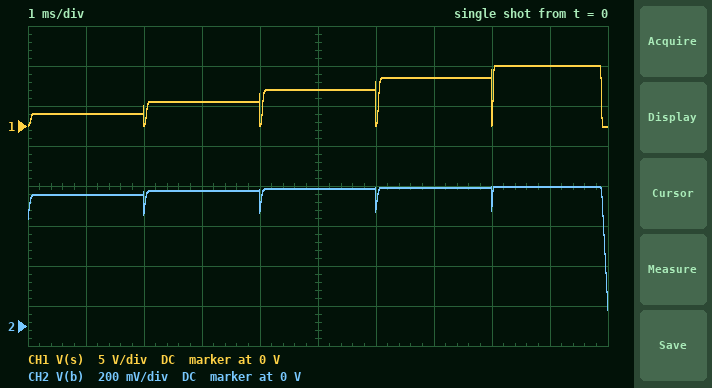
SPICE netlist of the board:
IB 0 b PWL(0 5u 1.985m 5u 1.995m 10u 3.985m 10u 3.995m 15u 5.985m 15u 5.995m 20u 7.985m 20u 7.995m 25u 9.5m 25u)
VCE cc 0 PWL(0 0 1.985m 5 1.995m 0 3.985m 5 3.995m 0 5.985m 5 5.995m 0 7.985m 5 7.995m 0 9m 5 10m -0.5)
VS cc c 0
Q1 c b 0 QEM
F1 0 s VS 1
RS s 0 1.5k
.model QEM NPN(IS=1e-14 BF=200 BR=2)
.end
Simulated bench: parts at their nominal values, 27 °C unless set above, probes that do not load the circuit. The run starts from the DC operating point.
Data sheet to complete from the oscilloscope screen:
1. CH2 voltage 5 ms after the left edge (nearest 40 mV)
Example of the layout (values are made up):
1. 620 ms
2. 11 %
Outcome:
1. 680 mV
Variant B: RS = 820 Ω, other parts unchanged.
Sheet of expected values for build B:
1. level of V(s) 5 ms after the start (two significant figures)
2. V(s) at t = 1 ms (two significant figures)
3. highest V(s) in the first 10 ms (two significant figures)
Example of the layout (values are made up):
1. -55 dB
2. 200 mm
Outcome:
1. 2.5 V
2. 820 mV
3. 4.1 V
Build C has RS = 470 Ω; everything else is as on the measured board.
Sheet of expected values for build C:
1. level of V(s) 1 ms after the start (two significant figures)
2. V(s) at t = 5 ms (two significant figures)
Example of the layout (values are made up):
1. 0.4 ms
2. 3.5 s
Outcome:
1. 470 mV
2. 1.4 V
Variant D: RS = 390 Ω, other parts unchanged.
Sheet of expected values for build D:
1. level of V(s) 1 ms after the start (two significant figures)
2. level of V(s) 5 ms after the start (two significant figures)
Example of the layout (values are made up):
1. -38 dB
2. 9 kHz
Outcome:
1. 390 mV
2. 1.2 V
